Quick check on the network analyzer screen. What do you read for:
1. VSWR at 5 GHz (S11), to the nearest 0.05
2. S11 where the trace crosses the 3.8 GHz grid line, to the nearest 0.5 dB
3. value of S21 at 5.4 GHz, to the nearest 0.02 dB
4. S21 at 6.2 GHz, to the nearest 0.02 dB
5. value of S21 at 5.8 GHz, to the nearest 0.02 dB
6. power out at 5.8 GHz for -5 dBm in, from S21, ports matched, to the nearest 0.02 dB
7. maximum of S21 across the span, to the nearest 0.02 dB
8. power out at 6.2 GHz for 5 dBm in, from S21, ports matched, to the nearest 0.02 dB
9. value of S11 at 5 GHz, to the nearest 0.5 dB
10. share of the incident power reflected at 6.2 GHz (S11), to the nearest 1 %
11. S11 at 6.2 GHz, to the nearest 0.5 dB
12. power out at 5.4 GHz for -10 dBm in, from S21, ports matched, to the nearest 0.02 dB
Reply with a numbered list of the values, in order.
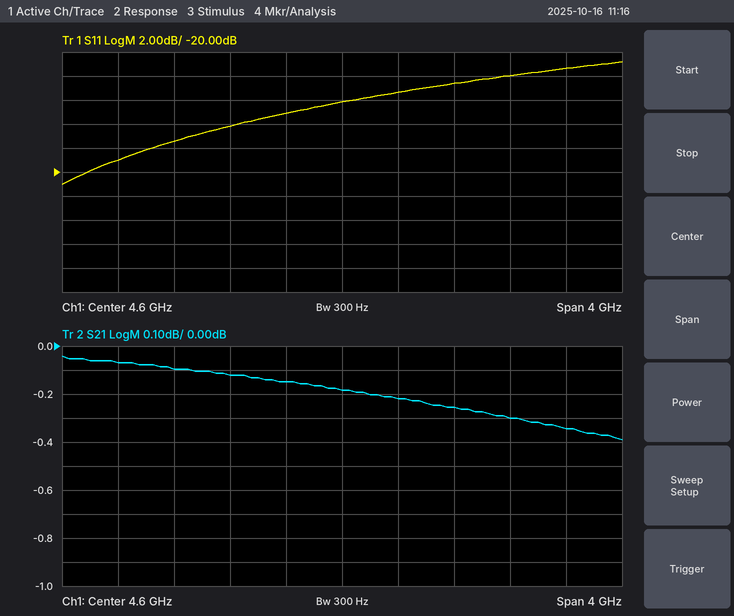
1. 1.55
2. -16.0 dB
3. -0.26 dB
4. -0.34 dB
5. -0.30 dB
6. -5.30 dBm
7. -0.04 dB
8. 4.66 dBm
9. -13.5 dB
10. 7 %
11. -11.5 dB
12. -10.26 dBm
